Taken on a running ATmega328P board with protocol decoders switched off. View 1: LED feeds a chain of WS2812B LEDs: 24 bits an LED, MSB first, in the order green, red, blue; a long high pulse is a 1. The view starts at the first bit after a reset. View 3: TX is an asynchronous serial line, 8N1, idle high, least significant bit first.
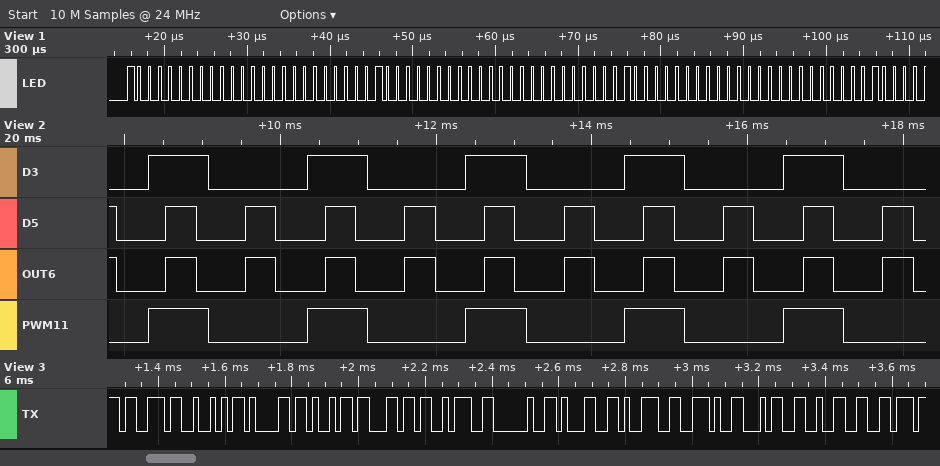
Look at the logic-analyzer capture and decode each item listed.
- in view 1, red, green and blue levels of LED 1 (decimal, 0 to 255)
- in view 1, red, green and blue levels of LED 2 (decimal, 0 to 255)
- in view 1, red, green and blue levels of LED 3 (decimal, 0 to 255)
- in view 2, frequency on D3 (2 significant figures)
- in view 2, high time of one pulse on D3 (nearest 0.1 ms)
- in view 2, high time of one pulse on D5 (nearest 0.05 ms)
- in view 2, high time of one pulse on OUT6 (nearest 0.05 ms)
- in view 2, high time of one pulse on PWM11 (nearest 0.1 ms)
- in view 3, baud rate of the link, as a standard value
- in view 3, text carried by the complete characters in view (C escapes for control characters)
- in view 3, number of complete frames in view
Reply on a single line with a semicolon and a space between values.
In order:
0, 128, 0; 0, 128, 0; 0, 128, 0; 490 Hz; 0.8 ms; 0.40 ms; 0.40 ms; 0.8 ms; 57600 baud; "sRail: 19.42v"; 13
